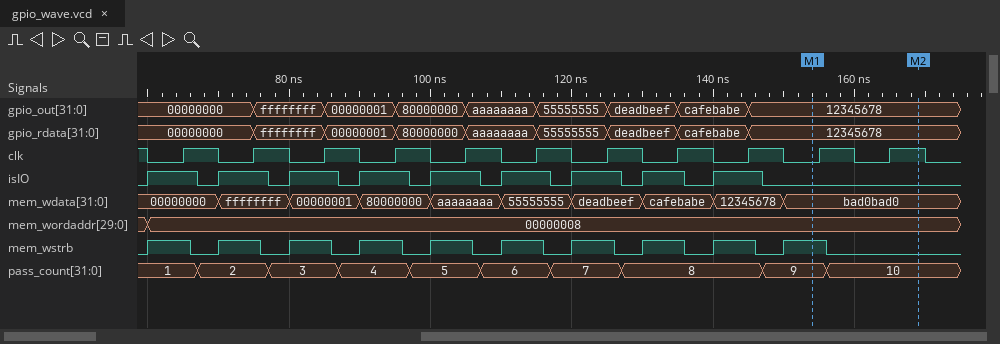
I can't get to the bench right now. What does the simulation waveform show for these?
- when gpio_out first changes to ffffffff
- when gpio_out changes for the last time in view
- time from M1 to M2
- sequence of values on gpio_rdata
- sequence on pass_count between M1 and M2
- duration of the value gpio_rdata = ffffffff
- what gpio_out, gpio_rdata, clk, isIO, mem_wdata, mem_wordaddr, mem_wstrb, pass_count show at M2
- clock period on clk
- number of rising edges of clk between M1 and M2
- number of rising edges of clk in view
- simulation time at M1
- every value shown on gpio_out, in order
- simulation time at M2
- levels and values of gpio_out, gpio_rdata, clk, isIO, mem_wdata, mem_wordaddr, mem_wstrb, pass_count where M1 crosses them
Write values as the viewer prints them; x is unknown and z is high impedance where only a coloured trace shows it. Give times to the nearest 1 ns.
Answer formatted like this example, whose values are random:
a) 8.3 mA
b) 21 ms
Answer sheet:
a) 75 ns
b) 145 ns
c) 15 ns
d) 00000000, ffffffff, 00000001, 80000000, aaaaaaaa, 55555555, deadbeef, cafebabe, 12345678
e) 9, 10
f) 10 ns
g) gpio_out=12345678, gpio_rdata=12345678, clk=1, isIO=0, mem_wdata=bad0bad0, mem_wordaddr=00000008, mem_wstrb=0, pass_count=10
h) 10 ns
i) 2
j) 11
k) 154 ns
l) 00000000, ffffffff, 00000001, 80000000, aaaaaaaa, 55555555, deadbeef, cafebabe, 12345678
m) 169 ns
n) gpio_out=12345678, gpio_rdata=12345678, clk=0, isIO=0, mem_wdata=bad0bad0, mem_wordaddr=00000008, mem_wstrb=1, pass_count=9
